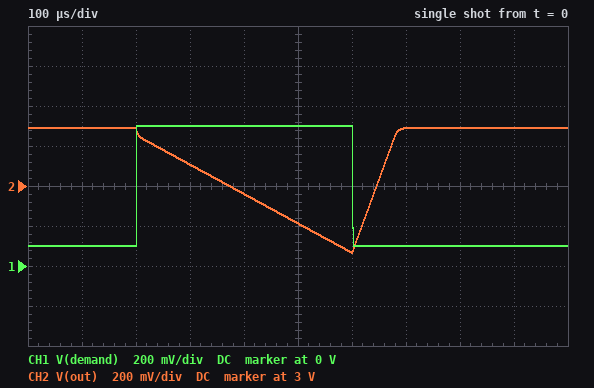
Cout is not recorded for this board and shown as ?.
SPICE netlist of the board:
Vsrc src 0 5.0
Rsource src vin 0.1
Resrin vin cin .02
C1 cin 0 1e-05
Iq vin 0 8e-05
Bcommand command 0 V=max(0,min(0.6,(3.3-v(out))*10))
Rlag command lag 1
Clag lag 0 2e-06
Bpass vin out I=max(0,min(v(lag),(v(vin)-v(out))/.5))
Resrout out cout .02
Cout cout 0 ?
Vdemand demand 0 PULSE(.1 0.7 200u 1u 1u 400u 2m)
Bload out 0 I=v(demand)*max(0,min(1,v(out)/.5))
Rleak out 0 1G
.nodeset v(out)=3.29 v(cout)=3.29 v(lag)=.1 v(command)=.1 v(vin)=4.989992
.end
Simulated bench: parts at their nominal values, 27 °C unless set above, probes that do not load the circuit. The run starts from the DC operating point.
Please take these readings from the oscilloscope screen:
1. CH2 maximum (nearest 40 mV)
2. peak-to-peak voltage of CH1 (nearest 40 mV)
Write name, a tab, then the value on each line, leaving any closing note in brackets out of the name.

CH2 maximum	3.28 V
peak-to-peak voltage of CH1	600 mV
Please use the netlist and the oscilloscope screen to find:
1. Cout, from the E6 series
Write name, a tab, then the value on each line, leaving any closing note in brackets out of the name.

Cout, from the E6 series	68 µF
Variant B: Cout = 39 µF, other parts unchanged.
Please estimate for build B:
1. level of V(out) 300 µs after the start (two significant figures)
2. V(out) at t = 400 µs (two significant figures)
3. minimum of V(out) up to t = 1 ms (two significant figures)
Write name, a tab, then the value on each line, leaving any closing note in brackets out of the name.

level of V(out) 300 µs after the start	3.0 V
V(out) at t = 400 µs	2.7 V
minimum of V(out) up to t = 1 ms	2.2 V
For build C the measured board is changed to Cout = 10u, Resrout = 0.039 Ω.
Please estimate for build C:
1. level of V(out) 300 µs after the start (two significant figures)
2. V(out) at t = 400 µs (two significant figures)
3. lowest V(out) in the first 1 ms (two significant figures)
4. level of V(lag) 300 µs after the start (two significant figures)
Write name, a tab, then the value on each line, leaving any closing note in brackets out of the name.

level of V(out) 300 µs after the start	2.2 V
V(out) at t = 400 µs	1.2 V
lowest V(out) in the first 1 ms	430 mV
level of V(lag) 300 µs after the start	600 mV
